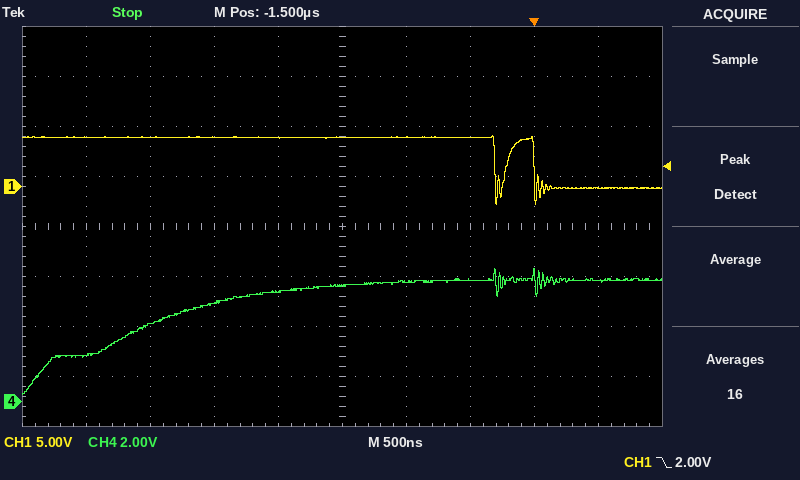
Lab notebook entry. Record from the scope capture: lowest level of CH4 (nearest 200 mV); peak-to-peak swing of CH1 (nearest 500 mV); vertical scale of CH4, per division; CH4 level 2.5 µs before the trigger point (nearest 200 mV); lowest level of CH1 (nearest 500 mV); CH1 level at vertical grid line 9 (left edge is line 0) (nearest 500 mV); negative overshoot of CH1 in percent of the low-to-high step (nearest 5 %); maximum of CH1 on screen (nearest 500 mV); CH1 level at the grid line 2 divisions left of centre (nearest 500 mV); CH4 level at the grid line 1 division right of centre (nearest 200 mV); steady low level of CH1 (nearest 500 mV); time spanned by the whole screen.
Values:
200 mV
7.0 V
2 V
4.0 V
-2.0 V
0.0 V
35 %
5.0 V
5.0 V
4.8 V
0.0 V
5 µs
